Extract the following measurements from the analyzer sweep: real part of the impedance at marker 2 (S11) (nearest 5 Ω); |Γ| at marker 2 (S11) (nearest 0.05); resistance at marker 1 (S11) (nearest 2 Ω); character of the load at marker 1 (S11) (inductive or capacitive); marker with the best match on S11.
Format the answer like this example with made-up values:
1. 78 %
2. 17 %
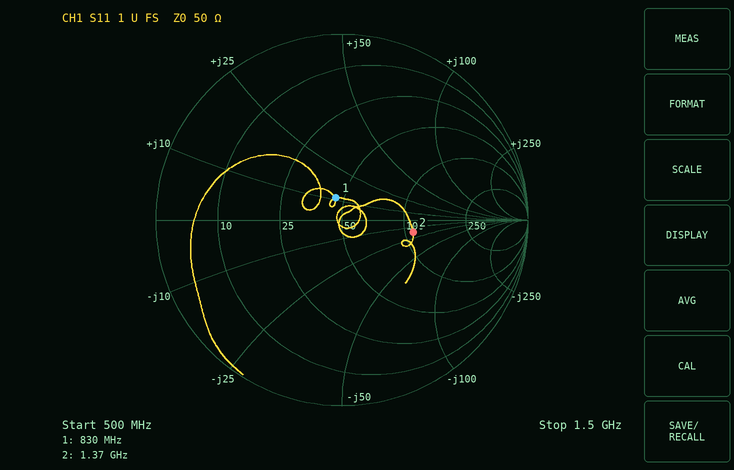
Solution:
1. 110 Ω
2. 0.40
3. 46 Ω
4. inductive
5. marker 1
